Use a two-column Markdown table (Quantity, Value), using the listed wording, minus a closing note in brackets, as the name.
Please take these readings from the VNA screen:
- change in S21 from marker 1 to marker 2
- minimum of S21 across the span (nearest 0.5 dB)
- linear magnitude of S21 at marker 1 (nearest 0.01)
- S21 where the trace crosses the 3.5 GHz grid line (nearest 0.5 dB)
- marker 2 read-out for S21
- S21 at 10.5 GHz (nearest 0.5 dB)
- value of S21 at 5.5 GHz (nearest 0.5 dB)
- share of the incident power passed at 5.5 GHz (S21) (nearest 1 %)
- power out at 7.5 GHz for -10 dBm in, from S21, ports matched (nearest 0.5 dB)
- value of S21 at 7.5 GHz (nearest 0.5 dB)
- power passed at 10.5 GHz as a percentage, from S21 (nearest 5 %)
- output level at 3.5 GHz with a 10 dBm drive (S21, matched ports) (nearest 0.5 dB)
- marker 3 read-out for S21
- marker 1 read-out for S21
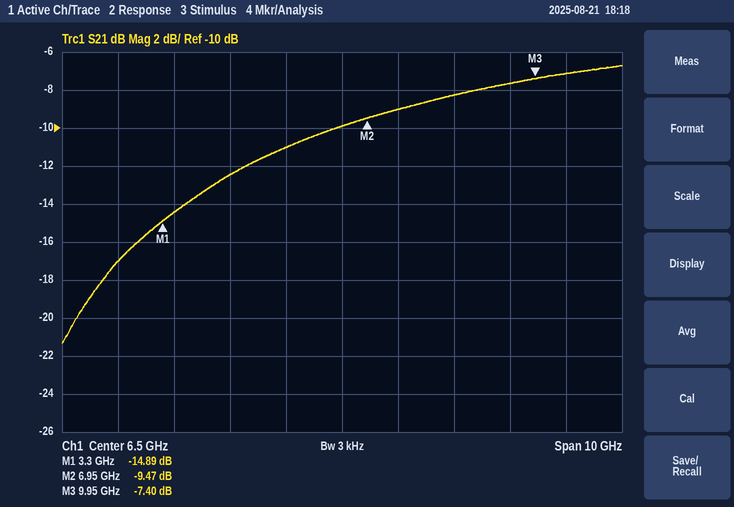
| Quantity | Value |
|---|---|
| change in S21 from marker 1 to marker 2 | 5.42 dB |
| minimum of S21 across the span | -21.5 dB |
| linear magnitude of S21 at marker 1 | 0.18 |
| S21 where the trace crosses the 3.5 GHz grid line | -14.5 dB |
| marker 2 read-out for S21 | -9.47 dB |
| S21 at 10.5 GHz | -7.0 dB |
| value of S21 at 5.5 GHz | -11.0 dB |
| share of the incident power passed at 5.5 GHz (S21) | 8 % |
| power out at 7.5 GHz for -10 dBm in, from S21, ports matched | -19.0 dBm |
| value of S21 at 7.5 GHz | -9.0 dB |
| power passed at 10.5 GHz as a percentage, from S21 | 20 % |
| output level at 3.5 GHz with a 10 dBm drive (S21, matched ports) | -4.5 dBm |
| marker 3 read-out for S21 | -7.40 dB |
| marker 1 read-out for S21 | -14.89 dB |
